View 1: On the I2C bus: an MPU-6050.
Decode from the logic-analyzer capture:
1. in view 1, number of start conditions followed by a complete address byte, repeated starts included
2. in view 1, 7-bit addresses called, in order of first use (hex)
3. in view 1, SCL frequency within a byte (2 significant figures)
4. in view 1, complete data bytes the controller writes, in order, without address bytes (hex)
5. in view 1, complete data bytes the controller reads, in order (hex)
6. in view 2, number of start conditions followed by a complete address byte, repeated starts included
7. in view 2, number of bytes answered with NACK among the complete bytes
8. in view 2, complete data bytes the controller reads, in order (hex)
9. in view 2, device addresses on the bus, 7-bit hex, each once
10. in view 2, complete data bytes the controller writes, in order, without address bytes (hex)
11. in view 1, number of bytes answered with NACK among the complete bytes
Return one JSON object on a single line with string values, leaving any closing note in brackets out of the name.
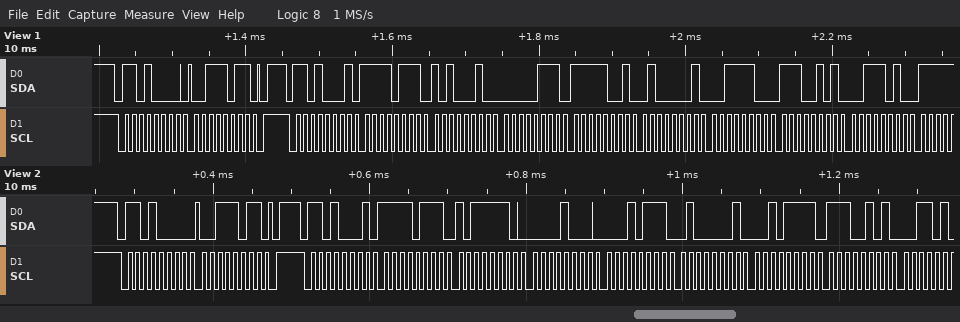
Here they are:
{"in view 1, number of start conditions followed by a complete address byte, repeated starts included": "2", "in view 1, 7-bit addresses called, in order of first use": "0x68", "in view 1, SCL frequency within a byte": "100 kHz", "in view 1, complete data bytes the controller writes, in order, without address bytes": "3B", "in view 1, complete data bytes the controller reads, in order": "F7 A2 07 F9 41 3C E5 3A", "in view 2, number of start conditions followed by a complete address byte, repeated starts included": "2", "in view 2, number of bytes answered with NACK among the complete bytes": "0", "in view 2, complete data bytes the controller reads, in order": "F7 BE 08 17 41 2F E5", "in view 2, device addresses on the bus, 7-bit hex, each once": "0x68", "in view 2, complete data bytes the controller writes, in order, without address bytes": "3B", "in view 1, number of bytes answered with NACK among the complete bytes": "0"}
